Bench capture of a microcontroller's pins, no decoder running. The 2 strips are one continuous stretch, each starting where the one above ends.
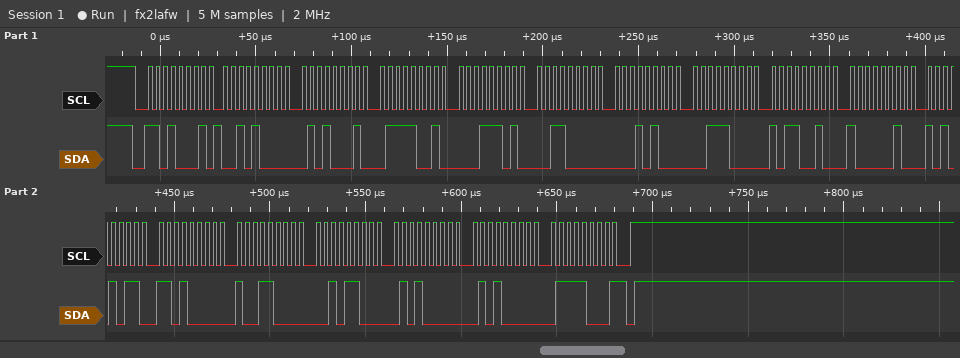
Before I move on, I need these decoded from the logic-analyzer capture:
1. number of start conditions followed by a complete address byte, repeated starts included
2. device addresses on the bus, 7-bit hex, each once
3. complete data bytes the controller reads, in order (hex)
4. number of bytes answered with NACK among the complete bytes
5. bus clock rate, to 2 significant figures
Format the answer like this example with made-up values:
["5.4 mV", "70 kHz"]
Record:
["1", "0x68", "28 51 79 1D 30 14 38 B2 82 AB D0 98 2C 50 50 78", "1", "250 kHz"]
